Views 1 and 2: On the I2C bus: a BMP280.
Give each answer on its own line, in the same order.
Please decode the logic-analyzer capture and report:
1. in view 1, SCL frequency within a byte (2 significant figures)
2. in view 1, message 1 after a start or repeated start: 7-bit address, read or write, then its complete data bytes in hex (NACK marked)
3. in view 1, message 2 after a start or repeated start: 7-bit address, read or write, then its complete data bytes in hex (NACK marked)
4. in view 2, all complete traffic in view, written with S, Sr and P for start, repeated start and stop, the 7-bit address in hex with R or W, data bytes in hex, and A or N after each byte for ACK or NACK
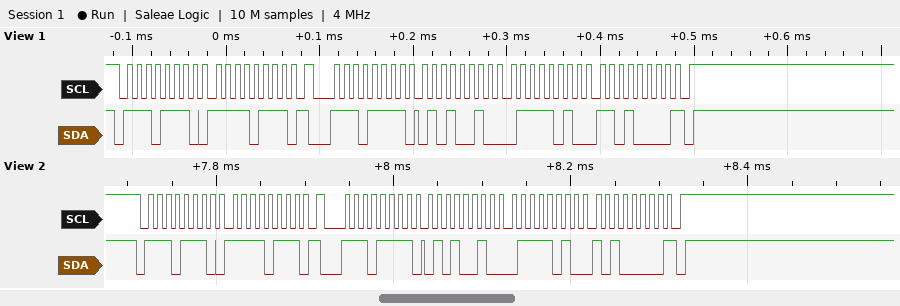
100 kHz
0x77 write: F7
0x77 read: 52 7A D0 NACK
S 77W A F7 A Sr 77R A 52 A 7A A A0 N P
